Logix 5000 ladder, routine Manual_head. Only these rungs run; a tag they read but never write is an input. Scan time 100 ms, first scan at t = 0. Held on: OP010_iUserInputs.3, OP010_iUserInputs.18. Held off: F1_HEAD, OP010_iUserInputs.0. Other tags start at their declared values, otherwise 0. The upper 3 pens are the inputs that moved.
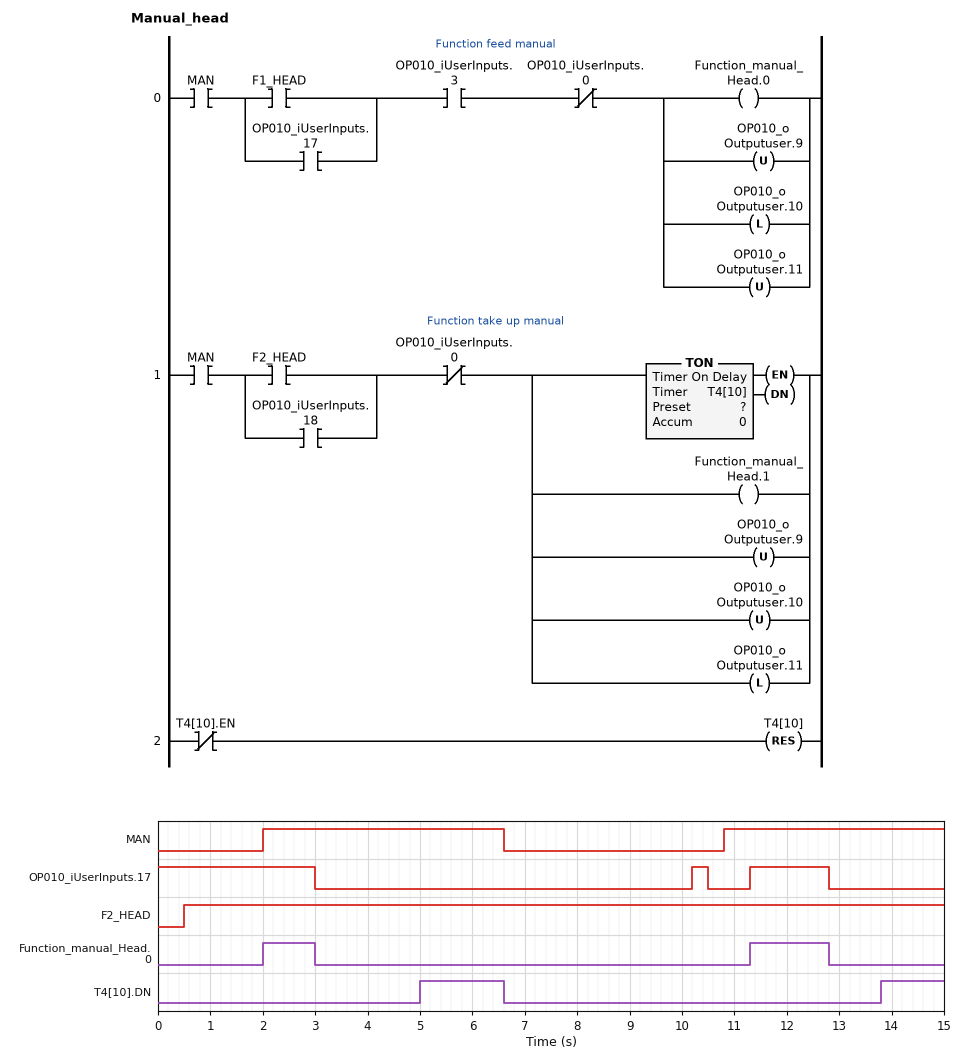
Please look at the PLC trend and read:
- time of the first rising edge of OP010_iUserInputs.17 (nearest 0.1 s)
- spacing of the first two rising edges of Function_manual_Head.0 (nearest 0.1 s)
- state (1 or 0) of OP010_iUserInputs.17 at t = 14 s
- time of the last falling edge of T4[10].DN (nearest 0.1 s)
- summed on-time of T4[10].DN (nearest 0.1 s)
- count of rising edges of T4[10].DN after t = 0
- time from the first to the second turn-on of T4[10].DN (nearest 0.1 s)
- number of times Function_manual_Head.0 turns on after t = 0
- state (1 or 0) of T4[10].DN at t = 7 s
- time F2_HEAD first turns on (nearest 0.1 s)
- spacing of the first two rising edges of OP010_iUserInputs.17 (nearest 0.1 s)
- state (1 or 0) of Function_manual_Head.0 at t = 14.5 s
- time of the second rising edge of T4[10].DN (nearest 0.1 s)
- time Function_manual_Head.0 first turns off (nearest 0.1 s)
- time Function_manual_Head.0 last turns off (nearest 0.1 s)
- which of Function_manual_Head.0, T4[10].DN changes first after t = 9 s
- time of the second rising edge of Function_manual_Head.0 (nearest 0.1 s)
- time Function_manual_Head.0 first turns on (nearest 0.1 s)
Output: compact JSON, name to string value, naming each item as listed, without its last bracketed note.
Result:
{"time of the first rising edge of OP010_iUserInputs.17": "10.2 s", "spacing of the first two rising edges of Function_manual_Head.0": "9.3 s", "state (1 or 0) of OP010_iUserInputs.17 at t = 14 s": "0", "time of the last falling edge of T4[10].DN": "6.6 s", "summed on-time of T4[10].DN": "2.8 s", "count of rising edges of T4[10].DN after t = 0": "2", "time from the first to the second turn-on of T4[10].DN": "8.8 s", "number of times Function_manual_Head.0 turns on after t = 0": "2", "state (1 or 0) of T4[10].DN at t = 7 s": "0", "time F2_HEAD first turns on": "0.5 s", "spacing of the first two rising edges of OP010_iUserInputs.17": "1.1 s", "state (1 or 0) of Function_manual_Head.0 at t = 14.5 s": "0", "time of the second rising edge of T4[10].DN": "13.8 s", "time Function_manual_Head.0 first turns off": "3.0 s", "time Function_manual_Head.0 last turns off": "12.8 s", "which of Function_manual_Head.0, T4[10].DN changes first after t = 9 s": "Function_manual_Head.0", "time of the second rising edge of Function_manual_Head.0": "11.3 s", "time Function_manual_Head.0 first turns on": "2.0 s"}
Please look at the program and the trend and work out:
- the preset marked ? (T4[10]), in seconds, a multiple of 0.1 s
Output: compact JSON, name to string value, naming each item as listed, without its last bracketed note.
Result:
{"the preset marked ? (T4[10]), in seconds, a multiple of 0.1 s": "3.0 s"}
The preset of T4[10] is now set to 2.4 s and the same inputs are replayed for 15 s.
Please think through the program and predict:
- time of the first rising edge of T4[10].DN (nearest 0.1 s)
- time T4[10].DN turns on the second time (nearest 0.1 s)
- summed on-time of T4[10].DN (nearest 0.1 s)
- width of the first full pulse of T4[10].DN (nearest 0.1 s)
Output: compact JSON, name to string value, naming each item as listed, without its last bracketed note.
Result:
{"time of the first rising edge of T4[10].DN": "4.4 s", "time T4[10].DN turns on the second time": "13.2 s", "summed on-time of T4[10].DN": "4.0 s", "width of the first full pulse of T4[10].DN": "2.2 s"}
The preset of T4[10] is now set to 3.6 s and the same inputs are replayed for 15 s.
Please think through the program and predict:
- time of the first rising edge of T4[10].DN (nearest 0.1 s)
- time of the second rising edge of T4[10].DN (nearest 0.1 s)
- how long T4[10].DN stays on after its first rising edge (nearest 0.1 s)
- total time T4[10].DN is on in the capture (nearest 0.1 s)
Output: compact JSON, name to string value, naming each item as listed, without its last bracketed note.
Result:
{"time of the first rising edge of T4[10].DN": "5.6 s", "time of the second rising edge of T4[10].DN": "14.4 s", "how long T4[10].DN stays on after its first rising edge": "1.0 s", "total time T4[10].DN is on in the capture": "1.6 s"}
